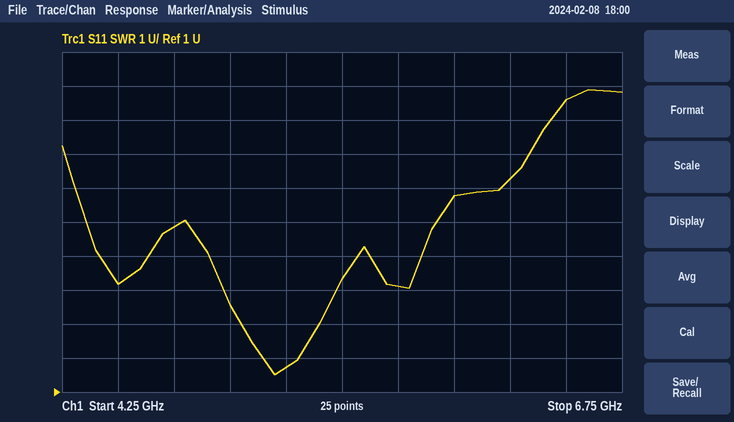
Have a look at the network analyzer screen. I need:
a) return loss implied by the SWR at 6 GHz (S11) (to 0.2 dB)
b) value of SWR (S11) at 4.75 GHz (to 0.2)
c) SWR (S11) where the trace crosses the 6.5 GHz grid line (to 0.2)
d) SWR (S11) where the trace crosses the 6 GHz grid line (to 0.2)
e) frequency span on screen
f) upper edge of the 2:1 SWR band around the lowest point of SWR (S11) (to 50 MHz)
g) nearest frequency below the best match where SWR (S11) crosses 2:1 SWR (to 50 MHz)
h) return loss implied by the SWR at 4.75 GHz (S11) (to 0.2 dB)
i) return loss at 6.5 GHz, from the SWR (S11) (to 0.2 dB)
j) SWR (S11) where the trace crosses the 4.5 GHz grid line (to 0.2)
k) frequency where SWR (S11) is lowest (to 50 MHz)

2.6 dB
5.8
9.6
6.8
2.5 GHz
5.30 GHz
5.15 GHz
3.0 dB
1.8 dB
4.2
5.20 GHz
